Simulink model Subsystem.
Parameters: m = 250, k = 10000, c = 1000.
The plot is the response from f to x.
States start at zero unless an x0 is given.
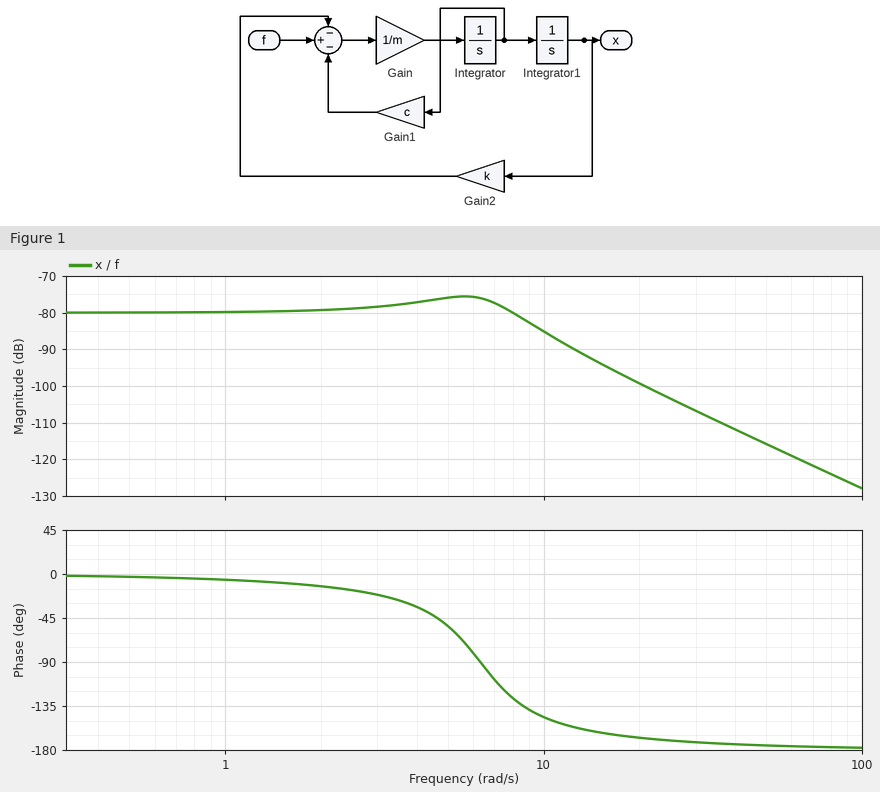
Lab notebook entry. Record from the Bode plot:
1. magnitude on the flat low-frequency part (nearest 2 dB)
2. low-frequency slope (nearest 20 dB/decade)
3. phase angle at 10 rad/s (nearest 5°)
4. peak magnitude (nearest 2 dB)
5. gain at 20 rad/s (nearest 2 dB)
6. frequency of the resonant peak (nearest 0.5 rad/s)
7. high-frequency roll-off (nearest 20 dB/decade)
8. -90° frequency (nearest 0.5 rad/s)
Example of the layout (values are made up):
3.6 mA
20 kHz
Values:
-80 dB
0 dB/decade
-145°
-76 dB
-100 dB
5.5 rad/s
-40 dB/decade
6.5 rad/s
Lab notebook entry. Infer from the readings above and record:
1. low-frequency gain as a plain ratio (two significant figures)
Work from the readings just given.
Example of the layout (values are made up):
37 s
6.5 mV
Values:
0.00010
